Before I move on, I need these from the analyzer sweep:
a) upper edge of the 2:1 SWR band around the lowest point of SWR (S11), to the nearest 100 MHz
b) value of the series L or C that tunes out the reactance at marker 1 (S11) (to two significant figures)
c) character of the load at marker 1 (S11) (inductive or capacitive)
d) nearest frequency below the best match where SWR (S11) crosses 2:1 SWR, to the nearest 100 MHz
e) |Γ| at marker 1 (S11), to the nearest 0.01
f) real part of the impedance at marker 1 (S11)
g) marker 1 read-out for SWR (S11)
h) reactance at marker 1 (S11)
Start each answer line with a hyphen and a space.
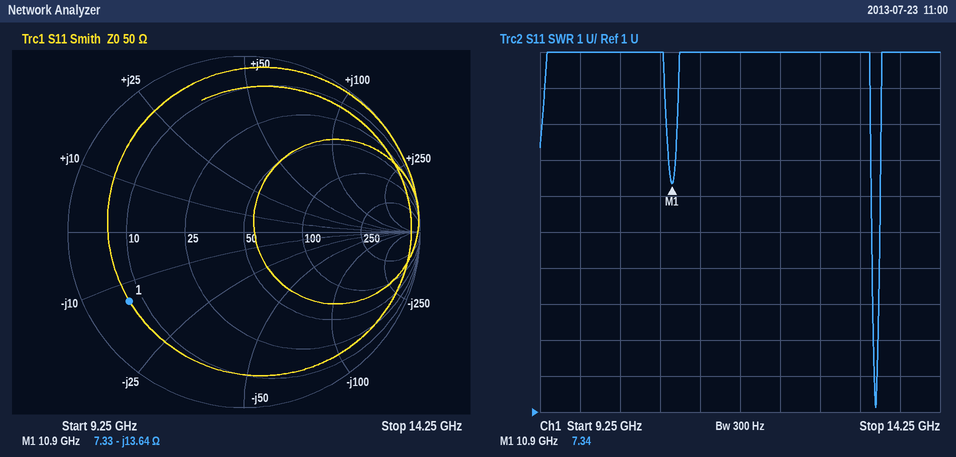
- 13.5 GHz
- 200 pH
- capacitive
- 13.4 GHz
- 0.76
- 7.33 Ω
- 7.34
- -13.64 Ω
